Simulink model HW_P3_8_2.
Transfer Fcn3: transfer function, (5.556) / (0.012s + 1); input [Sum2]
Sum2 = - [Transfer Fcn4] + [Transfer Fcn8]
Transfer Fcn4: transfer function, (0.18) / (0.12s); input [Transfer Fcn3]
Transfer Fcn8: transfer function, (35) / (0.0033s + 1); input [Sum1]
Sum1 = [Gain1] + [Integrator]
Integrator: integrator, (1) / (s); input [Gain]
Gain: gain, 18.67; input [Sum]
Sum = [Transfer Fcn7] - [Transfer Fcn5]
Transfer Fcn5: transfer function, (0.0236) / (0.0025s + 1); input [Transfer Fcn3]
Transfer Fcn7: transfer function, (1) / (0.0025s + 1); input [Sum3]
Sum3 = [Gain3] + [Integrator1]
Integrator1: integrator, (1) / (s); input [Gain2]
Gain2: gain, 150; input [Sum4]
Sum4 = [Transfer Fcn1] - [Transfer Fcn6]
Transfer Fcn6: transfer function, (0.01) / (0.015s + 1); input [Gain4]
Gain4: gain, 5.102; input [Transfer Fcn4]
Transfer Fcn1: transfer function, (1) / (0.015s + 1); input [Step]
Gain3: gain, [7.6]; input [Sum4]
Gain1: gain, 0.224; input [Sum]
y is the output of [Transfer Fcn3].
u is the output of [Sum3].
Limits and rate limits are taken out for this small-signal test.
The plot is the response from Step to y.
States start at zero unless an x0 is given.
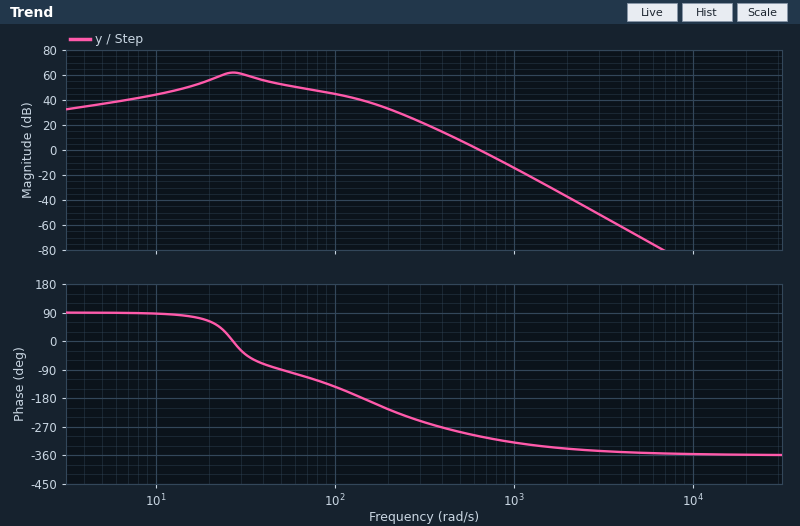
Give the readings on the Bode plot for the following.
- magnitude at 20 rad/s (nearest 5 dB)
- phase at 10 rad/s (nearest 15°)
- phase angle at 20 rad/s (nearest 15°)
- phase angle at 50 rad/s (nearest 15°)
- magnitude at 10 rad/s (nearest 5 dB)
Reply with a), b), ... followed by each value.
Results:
a) 55 dB
b) 90°
c) 60°
d) -90°
e) 45 dB
